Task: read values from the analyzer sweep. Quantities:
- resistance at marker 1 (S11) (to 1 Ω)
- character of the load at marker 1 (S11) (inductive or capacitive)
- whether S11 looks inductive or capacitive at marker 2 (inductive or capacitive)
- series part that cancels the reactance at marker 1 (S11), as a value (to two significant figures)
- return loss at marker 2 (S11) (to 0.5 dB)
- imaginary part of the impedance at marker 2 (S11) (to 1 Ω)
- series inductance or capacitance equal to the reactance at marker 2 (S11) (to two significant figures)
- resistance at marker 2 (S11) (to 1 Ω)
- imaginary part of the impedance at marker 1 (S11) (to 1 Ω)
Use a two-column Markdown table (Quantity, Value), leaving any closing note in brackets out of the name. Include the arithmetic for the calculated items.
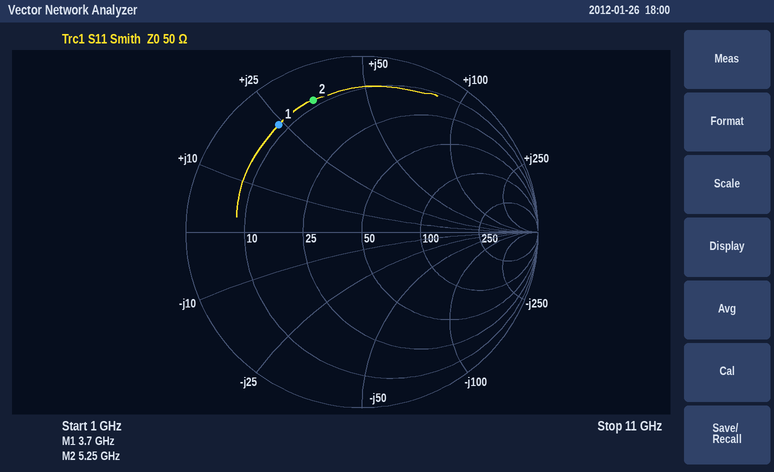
| Quantity | Value |
|---|---|
| resistance at marker 1 (S11) | 8 Ω |
| character of the load at marker 1 (S11) | inductive |
| whether S11 looks inductive or capacitive at marker 2 | inductive |
| series part that cancels the reactance at marker 1 (S11), as a value | C = 1/(2π × 3.7 GHz × 24 Ω) ≈ 1.8 pF |
| return loss at marker 2 (S11) | 2.0 dB |
| imaginary part of the impedance at marker 2 (S11) | +34 Ω |
| series inductance or capacitance equal to the reactance at marker 2 (S11) | L = 34 Ω/(2π × 5.25 GHz) ≈ 1.0 nH |
| resistance at marker 2 (S11) | 8 Ω |
| imaginary part of the impedance at marker 1 (S11) | +24 Ω |
